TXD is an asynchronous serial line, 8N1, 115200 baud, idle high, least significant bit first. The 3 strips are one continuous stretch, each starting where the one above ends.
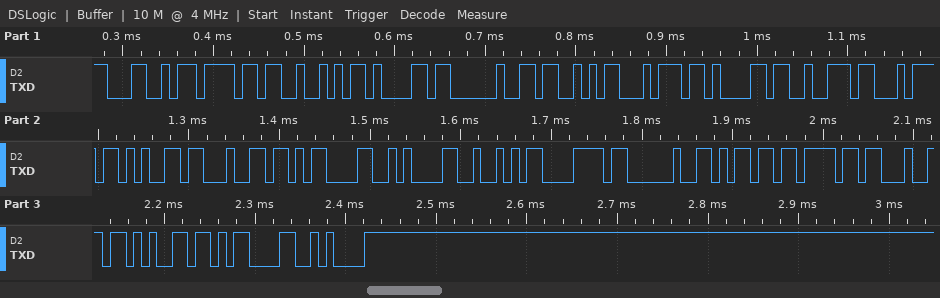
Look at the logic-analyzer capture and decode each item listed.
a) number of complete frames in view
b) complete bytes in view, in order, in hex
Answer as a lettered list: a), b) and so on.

a) 23
b) 4C 6F 52 61 20 53 74 61 72 74 65 64 0D 0A 52 78 20 6D 6F 64 65 0D 0A
